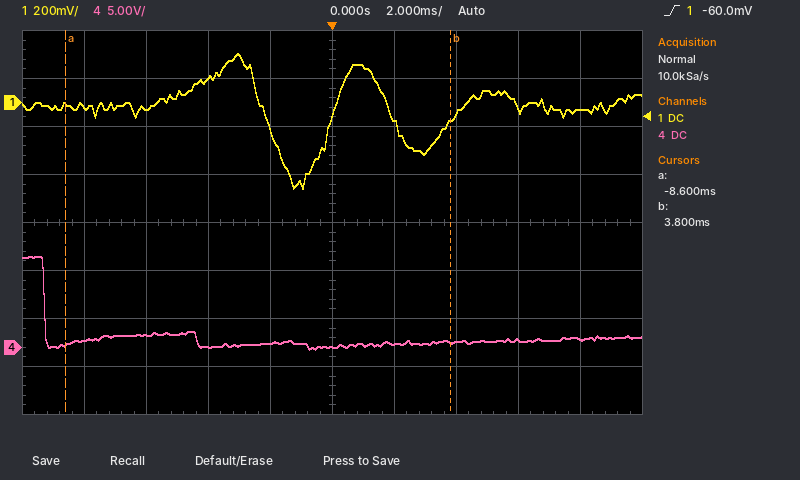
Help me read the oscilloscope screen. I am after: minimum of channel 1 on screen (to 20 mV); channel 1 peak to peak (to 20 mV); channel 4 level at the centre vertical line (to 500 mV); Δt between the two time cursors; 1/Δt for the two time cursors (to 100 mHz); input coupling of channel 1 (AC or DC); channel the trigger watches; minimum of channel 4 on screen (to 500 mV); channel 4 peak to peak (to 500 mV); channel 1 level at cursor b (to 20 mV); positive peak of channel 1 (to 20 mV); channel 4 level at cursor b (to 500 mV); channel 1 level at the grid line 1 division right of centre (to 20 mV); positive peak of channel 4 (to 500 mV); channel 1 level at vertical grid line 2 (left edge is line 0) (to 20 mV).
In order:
-360 mV
560 mV
0.0 V
12.4 ms
80.6 Hz
DC
channel 1
0.0 V
9.5 V
-80 mV
200 mV
500 mV
-80 mV
9.5 V
-20 mV
